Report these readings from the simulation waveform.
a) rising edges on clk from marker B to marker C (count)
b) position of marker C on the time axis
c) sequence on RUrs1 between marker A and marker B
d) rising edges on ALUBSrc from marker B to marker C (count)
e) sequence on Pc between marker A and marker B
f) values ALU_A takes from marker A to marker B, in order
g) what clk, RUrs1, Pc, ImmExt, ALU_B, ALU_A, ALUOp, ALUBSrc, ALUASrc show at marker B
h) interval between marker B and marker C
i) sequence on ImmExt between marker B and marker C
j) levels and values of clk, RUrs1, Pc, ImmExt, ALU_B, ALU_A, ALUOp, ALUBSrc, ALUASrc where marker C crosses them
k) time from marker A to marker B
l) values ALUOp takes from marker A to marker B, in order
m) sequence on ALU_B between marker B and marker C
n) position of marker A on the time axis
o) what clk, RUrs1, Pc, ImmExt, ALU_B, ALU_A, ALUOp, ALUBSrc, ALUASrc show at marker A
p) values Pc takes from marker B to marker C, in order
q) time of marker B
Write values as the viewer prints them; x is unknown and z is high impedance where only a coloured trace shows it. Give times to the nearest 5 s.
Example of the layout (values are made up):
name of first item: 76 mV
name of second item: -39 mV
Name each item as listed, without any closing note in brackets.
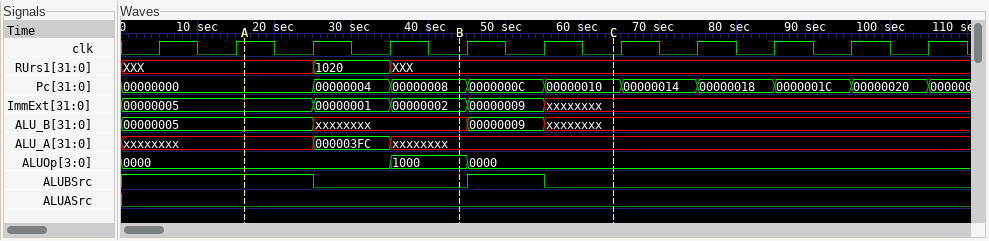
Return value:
rising edges on clk from marker B to marker C: 2
position of marker C on the time axis: 65 s
sequence on RUrs1 between marker A and marker B: XXX, 1020, XXX
rising edges on ALUBSrc from marker B to marker C: 1
sequence on Pc between marker A and marker B: 00000000, 00000004, 00000008
values ALU_A takes from marker A to marker B, in order: xxxxxxxx, 000003FC, xxxxxxxx
what clk, RUrs1, Pc, ImmExt, ALU_B, ALU_A, ALUOp, ALUBSrc, ALUASrc show at marker B: clk=0, RUrs1=XXX, Pc=00000008, ImmExt=00000002, ALU_B=xxxxxxxx, ALU_A=xxxxxxxx, ALUOp=1000, ALUBSrc=0, ALUASrc=0
interval between marker B and marker C: 20 s
sequence on ImmExt between marker B and marker C: 00000002, 00000009, xxxxxxxx
levels and values of clk, RUrs1, Pc, ImmExt, ALU_B, ALU_A, ALUOp, ALUBSrc, ALUASrc where marker C crosses them: clk=0, RUrs1=XXX, Pc=00000010, ImmExt=xxxxxxxx, ALU_B=xxxxxxxx, ALU_A=xxxxxxxx, ALUOp=0000, ALUBSrc=0, ALUASrc=0
time from marker A to marker B: 30 s
values ALUOp takes from marker A to marker B, in order: 0000, 1000
sequence on ALU_B between marker B and marker C: xxxxxxxx, 00000009, xxxxxxxx
position of marker A on the time axis: 15 s
what clk, RUrs1, Pc, ImmExt, ALU_B, ALU_A, ALUOp, ALUBSrc, ALUASrc show at marker A: clk=1, RUrs1=XXX, Pc=00000000, ImmExt=00000005, ALU_B=00000005, ALU_A=xxxxxxxx, ALUOp=0000, ALUBSrc=1, ALUASrc=0
values Pc takes from marker B to marker C, in order: 00000008, 0000000C, 00000010
time of marker B: 45 s
